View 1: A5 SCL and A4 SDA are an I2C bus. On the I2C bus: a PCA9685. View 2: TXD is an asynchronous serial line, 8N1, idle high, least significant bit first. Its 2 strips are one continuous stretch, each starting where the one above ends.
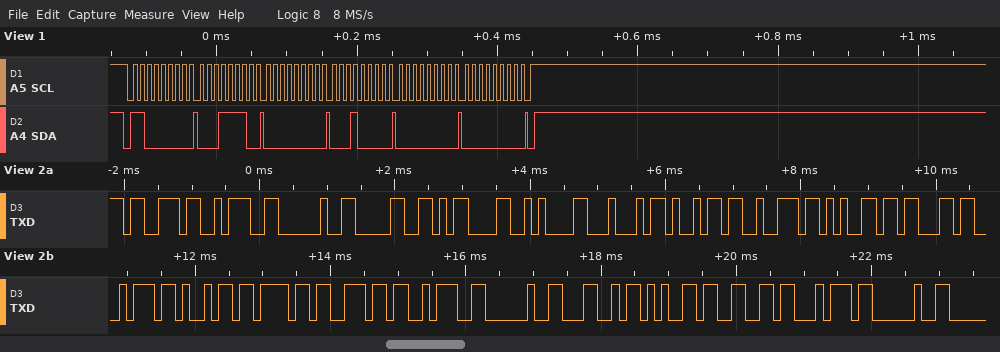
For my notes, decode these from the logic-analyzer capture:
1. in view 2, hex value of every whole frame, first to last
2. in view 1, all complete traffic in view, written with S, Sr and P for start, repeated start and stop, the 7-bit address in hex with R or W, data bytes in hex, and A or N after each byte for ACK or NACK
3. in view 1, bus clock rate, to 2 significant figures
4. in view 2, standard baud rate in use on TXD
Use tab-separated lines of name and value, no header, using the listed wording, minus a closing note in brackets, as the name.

in view 2, hex value of every whole frame, first to last	0x73 0x3A 0x20 0x30 0x0D 0x0A 0x44 0x69 0x72 0x65 0x63 0x74 0x69 0x6F 0x6E 0x3A 0x20 0x4C 0x65 0x66 0x74 0x20
in view 1, all complete traffic in view, written with S, Sr and P for start, repeated start and stop, the 7-bit address in hex with R or W, data bytes in hex, and A or N after each byte for ACK or NACK	S 60W A 1E A 00 A 10 A 00 A 00 A P
in view 1, bus clock rate, to 2 significant figures	100 kHz
in view 2, standard baud rate in use on TXD	9600 baud
